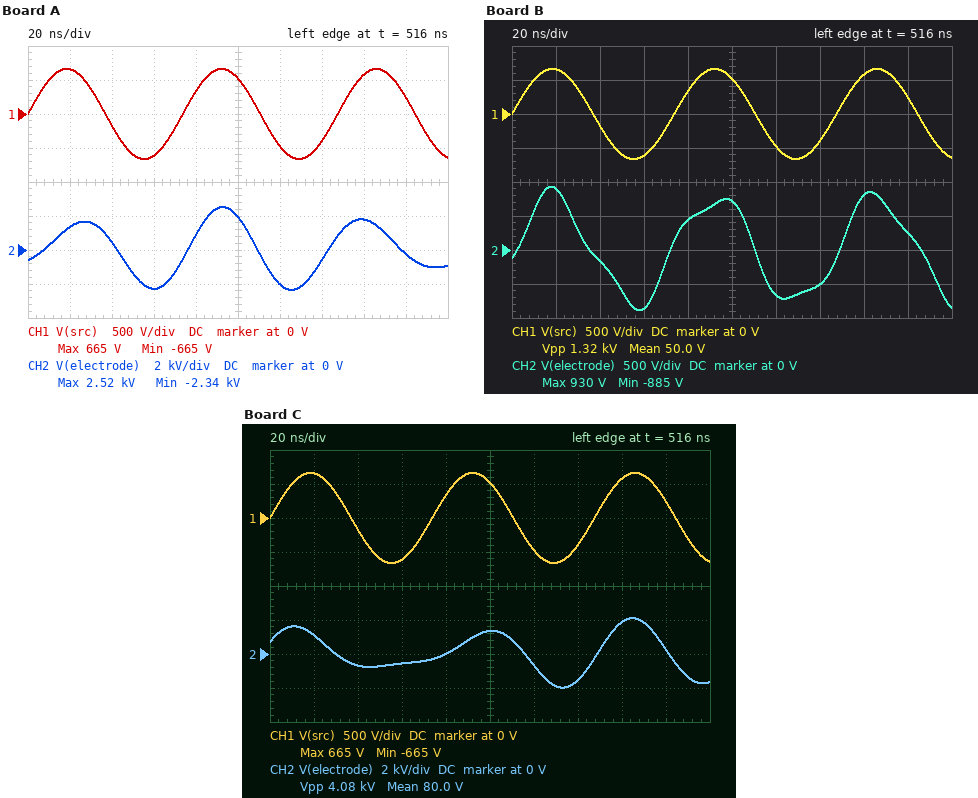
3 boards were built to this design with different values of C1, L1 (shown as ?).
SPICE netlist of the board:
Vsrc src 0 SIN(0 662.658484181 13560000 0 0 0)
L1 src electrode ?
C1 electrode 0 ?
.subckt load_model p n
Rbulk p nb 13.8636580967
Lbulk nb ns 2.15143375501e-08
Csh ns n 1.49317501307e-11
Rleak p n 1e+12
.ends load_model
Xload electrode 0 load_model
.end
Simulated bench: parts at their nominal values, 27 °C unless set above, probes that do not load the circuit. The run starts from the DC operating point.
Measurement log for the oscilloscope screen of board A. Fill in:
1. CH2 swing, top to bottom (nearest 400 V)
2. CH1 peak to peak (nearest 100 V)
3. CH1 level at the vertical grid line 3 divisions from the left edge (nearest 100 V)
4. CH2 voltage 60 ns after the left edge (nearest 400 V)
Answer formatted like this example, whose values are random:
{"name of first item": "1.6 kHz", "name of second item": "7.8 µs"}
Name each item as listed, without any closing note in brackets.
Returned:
{"CH2 swing, top to bottom": "4.8 kV", "CH1 peak to peak": "1.3 kV", "CH1 level at the vertical grid line 3 divisions from the left edge": "-600 V", "CH2 voltage 60 ns after the left edge": "-2.4 kV"}
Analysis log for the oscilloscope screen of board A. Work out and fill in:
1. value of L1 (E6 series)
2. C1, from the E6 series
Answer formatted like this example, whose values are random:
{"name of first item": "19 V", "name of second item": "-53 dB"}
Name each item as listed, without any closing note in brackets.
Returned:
{"value of L1": "2.2 µH", "C1, from the E6 series": "22 pF"}
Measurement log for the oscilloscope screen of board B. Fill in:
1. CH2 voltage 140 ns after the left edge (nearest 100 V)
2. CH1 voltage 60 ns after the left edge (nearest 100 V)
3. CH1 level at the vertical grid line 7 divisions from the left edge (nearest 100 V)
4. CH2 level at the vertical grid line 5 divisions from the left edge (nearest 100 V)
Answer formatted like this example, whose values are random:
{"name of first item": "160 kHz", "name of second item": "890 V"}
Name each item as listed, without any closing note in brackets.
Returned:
{"CH2 voltage 140 ns after the left edge": "-500 V", "CH1 voltage 60 ns after the left edge": "-600 V", "CH1 level at the vertical grid line 7 divisions from the left edge": "-400 V", "CH2 level at the vertical grid line 5 divisions from the left edge": "700 V"}
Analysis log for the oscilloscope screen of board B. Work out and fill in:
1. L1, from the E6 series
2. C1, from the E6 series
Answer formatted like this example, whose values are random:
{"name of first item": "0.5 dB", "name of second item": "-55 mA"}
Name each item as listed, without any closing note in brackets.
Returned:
{"L1, from the E6 series": "330 nH", "C1, from the E6 series": "47 pF"}
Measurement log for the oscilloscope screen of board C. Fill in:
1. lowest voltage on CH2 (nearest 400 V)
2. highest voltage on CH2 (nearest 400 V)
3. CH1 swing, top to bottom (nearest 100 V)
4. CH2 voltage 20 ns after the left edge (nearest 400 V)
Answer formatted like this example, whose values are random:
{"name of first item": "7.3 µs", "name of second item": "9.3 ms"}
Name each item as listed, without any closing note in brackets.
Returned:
{"lowest voltage on CH2": "-2.0 kV", "highest voltage on CH2": "2.0 kV", "CH1 swing, top to bottom": "1.3 kV", "CH2 voltage 20 ns after the left edge": "1.2 kV"}
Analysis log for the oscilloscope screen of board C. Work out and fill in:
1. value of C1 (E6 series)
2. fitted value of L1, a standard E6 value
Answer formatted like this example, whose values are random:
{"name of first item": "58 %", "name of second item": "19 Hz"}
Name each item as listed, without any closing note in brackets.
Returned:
{"value of C1": "33 pF", "fitted value of L1, a standard E6 value": "1.5 µH"}
